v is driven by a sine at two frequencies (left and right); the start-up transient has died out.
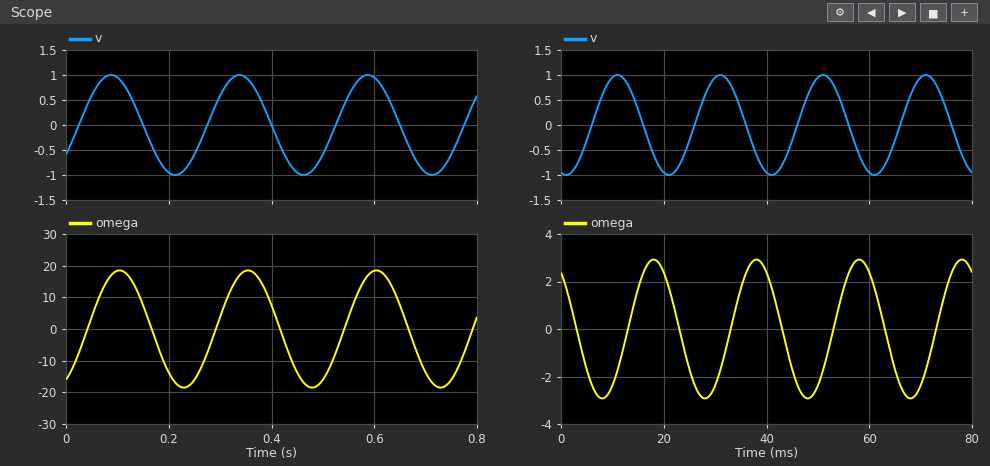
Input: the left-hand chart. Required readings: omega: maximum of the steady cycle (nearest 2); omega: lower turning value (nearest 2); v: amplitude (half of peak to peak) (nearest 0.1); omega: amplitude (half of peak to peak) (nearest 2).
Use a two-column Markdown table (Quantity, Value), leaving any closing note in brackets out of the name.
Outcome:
| Quantity | Value |
|---|---|
| omega: maximum of the steady cycle | 18 |
| omega: lower turning value | -18 |
| v: amplitude (half of peak to peak) | 1.0 |
| omega: amplitude (half of peak to peak) | 18 |
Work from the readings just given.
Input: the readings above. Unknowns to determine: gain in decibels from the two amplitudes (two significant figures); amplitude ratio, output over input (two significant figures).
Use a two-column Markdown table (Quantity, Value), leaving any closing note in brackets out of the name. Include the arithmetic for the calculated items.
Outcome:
| Quantity | Value |
|---|---|
| gain in decibels from the two amplitudes | 20 log10(18 / 1) = 25 dB |
| amplitude ratio, output over input | 18 / 1 = 18 |
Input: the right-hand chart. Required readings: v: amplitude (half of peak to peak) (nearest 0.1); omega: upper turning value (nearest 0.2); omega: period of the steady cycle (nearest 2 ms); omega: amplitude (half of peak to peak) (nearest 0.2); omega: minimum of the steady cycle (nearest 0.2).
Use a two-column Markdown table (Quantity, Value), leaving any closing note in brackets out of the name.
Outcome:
| Quantity | Value |
|---|---|
| v: amplitude (half of peak to peak) | 1.0 |
| omega: upper turning value | 3.0 |
| omega: period of the steady cycle | 20 ms |
| omega: amplitude (half of peak to peak) | 3.0 |
| omega: minimum of the steady cycle | -3.0 |
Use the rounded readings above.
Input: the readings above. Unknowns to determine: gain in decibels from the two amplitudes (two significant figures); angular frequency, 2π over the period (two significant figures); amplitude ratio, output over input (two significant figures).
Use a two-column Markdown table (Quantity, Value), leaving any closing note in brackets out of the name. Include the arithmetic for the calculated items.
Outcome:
| Quantity | Value |
|---|---|
| gain in decibels from the two amplitudes | 20 log10(3 / 1) = 9.5 dB |
| angular frequency, 2π over the period | 2π / 20 = 0.31 rad/ms |
| amplitude ratio, output over input | 3 / 1 = 3.0 |
